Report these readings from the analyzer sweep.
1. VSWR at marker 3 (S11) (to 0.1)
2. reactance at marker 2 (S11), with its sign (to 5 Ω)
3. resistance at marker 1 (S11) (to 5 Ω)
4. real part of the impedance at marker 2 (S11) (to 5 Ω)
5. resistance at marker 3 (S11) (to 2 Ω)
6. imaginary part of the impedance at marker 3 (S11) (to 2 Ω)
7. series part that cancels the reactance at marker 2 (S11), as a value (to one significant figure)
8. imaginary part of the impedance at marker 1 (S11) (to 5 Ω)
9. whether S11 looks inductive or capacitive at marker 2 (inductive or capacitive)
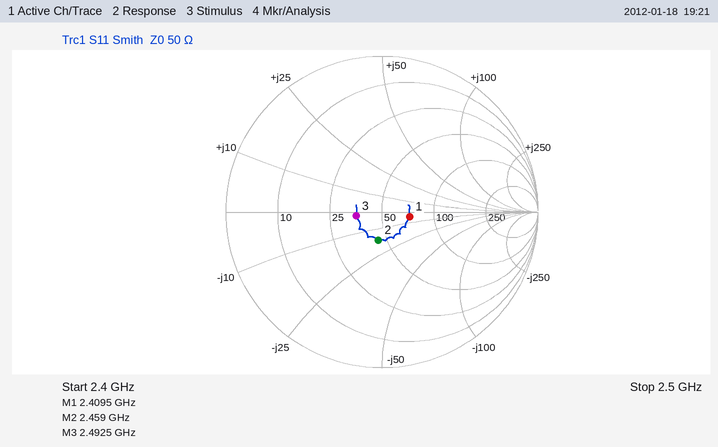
1.4
-15 Ω
70 Ω
45 Ω
36 Ω
-2 Ω
1 nH
-5 Ω
capacitive
